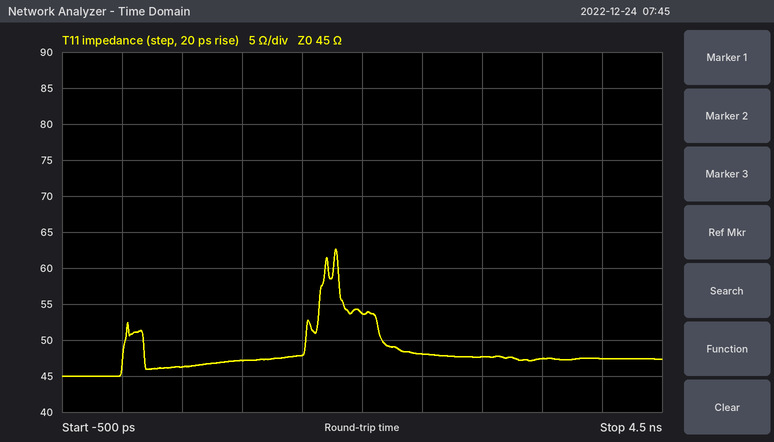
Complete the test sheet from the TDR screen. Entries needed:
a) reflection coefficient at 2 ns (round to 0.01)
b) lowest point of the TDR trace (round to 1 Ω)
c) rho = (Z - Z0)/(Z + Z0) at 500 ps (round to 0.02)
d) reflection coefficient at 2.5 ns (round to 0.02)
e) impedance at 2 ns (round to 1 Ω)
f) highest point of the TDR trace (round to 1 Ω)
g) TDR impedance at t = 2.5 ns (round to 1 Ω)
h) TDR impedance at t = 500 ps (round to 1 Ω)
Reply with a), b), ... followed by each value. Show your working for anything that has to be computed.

a) (54 − 45)/(54 + 45) ≈ +0.09
b) 45 Ω
c) (46 − 45)/(46 + 45) ≈ +0.0110, so +0.02 to the nearest 0.02
d) (48 − 45)/(48 + 45) ≈ +0.0323, so +0.04 to the nearest 0.02
e) 54 Ω
f) 63 Ω
g) 48 Ω
h) 46 Ω
